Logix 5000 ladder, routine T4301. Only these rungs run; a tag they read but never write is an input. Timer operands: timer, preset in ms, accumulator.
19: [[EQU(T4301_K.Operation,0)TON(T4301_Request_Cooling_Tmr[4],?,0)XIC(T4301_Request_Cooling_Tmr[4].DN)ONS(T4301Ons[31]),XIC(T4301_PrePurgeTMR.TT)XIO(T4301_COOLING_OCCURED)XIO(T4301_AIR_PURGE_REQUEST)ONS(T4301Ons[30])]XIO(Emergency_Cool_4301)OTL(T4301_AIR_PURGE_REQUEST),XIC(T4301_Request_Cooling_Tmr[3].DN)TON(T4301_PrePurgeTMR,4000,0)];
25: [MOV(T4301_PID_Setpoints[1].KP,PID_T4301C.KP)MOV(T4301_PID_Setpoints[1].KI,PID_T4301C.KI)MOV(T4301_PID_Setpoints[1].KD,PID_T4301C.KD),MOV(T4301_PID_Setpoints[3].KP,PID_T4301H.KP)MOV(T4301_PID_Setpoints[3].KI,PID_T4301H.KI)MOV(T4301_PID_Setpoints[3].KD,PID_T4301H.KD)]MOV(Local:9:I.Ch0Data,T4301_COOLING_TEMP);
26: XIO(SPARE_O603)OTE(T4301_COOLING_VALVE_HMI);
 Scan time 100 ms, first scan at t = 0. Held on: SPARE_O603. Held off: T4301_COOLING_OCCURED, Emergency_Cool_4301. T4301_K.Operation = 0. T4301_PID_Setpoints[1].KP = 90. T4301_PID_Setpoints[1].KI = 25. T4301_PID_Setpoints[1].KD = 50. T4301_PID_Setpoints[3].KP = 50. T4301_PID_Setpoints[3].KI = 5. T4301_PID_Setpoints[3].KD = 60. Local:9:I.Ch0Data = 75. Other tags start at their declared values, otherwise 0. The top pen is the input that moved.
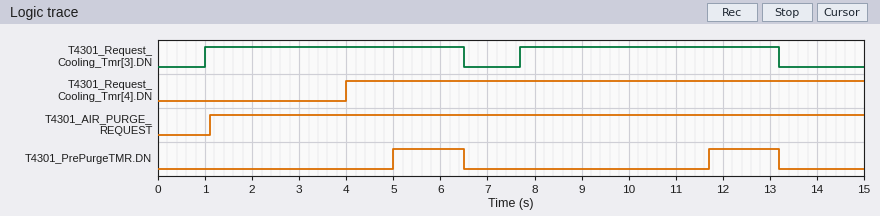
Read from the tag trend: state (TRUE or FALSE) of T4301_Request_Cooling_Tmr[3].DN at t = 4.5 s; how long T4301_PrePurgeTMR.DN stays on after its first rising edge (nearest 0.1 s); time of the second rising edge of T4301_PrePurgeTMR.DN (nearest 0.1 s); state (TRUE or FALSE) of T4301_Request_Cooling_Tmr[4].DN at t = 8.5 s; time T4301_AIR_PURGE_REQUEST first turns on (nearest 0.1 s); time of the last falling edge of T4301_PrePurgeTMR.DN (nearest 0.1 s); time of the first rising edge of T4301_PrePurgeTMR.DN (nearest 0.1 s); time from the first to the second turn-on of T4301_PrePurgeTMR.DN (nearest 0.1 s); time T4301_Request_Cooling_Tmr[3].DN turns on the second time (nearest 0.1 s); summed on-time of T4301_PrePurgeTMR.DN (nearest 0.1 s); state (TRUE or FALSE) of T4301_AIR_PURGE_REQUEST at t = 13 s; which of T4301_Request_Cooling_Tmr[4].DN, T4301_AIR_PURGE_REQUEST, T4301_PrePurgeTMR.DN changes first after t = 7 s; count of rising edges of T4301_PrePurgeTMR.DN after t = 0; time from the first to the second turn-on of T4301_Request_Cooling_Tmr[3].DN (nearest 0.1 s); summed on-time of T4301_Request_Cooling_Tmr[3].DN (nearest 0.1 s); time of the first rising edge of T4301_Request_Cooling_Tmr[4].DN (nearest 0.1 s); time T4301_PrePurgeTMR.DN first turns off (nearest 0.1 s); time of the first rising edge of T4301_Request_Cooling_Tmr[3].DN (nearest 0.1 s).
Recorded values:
TRUE
1.5 s
11.7 s
TRUE
1.1 s
13.2 s
5.0 s
6.7 s
7.7 s
3.0 s
TRUE
T4301_PrePurgeTMR.DN
2
6.7 s
11.0 s
4.0 s
6.5 s
1.0 s
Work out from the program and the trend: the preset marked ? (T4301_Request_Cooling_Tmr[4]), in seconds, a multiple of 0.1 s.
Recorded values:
4.0 s
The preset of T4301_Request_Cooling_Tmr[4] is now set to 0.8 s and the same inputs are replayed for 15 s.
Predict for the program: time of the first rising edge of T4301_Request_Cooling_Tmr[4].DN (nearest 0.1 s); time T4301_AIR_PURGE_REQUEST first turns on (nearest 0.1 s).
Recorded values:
0.8 s
0.8 s
